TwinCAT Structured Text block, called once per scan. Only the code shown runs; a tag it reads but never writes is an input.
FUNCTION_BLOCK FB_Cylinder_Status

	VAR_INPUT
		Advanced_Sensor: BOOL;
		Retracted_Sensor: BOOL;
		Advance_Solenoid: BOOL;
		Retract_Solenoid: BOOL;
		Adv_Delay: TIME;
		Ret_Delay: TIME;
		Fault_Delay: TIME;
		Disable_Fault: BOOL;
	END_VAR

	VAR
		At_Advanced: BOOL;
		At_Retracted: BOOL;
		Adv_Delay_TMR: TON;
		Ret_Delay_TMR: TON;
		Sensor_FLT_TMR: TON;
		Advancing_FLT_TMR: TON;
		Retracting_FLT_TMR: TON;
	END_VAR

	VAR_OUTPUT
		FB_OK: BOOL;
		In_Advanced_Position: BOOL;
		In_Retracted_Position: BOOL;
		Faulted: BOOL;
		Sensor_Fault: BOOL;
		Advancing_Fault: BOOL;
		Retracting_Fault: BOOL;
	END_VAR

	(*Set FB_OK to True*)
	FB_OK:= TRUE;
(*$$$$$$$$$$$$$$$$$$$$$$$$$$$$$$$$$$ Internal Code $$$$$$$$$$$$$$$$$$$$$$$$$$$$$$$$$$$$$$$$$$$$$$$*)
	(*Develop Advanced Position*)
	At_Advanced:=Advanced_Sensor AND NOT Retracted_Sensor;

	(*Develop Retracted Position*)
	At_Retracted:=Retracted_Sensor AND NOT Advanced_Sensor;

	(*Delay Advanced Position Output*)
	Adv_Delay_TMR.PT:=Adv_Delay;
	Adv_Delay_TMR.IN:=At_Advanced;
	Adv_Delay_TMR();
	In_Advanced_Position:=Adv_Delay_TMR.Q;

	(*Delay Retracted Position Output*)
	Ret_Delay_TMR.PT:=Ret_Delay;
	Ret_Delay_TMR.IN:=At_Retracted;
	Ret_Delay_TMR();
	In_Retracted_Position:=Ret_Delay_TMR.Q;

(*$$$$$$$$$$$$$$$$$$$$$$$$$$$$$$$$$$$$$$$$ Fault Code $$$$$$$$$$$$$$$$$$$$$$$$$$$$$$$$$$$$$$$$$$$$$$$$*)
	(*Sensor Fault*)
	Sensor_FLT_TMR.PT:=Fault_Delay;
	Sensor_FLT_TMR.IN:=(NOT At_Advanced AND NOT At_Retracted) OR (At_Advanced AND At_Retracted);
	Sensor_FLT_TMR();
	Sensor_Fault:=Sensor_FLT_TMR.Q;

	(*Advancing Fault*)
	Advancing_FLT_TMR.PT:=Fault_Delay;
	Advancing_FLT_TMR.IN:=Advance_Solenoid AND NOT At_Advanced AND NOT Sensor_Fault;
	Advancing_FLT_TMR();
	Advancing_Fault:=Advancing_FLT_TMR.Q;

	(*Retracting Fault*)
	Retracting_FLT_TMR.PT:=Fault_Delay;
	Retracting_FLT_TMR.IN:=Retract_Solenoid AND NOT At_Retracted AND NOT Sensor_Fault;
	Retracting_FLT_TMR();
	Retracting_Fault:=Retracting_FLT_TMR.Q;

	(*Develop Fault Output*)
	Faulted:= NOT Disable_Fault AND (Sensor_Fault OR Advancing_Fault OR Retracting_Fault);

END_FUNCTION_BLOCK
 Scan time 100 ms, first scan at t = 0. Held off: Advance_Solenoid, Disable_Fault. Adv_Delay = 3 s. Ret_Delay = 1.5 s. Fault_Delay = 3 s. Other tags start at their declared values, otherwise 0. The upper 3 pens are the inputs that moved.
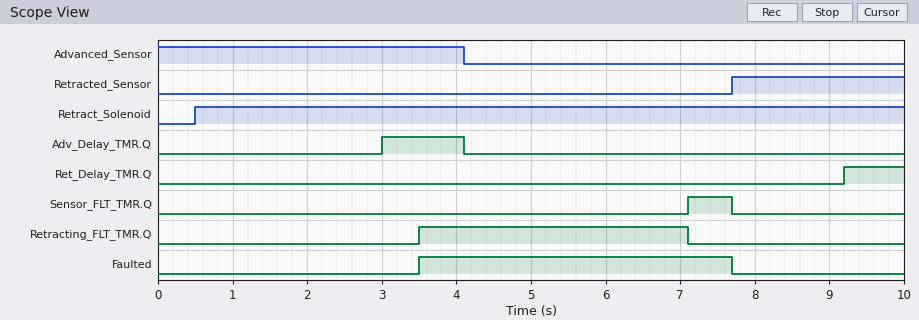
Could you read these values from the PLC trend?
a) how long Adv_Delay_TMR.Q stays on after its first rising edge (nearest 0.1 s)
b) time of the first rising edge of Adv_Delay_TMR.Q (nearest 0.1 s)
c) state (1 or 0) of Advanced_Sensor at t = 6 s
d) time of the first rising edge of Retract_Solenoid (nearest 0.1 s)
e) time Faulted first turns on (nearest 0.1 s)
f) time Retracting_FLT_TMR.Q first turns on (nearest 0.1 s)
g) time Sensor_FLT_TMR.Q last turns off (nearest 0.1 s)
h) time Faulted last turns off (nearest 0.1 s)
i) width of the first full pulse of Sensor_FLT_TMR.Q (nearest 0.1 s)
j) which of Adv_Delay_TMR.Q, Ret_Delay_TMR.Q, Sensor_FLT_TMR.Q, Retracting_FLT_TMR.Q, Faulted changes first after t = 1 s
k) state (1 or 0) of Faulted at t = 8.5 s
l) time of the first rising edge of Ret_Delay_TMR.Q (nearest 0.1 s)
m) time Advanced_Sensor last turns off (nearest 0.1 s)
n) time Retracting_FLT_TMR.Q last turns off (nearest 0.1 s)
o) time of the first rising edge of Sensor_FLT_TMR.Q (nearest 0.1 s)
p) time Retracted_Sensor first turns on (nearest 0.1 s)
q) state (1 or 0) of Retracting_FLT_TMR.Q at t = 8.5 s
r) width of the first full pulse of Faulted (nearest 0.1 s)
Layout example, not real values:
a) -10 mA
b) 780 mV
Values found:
a) 1.1 s
b) 3.0 s
c) 0
d) 0.5 s
e) 3.5 s
f) 3.5 s
g) 7.7 s
h) 7.7 s
i) 0.6 s
j) Adv_Delay_TMR.Q
k) 0
l) 9.2 s
m) 4.1 s
n) 7.1 s
o) 7.1 s
p) 7.7 s
q) 0
r) 4.2 s
